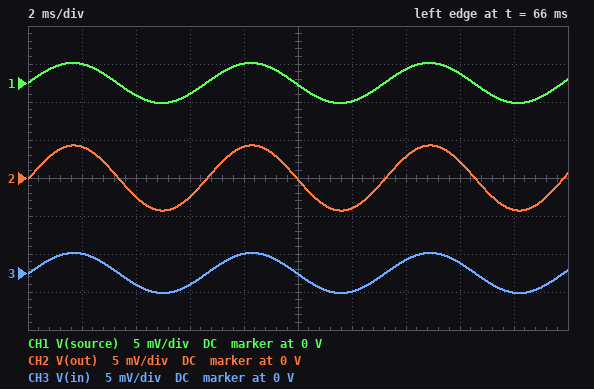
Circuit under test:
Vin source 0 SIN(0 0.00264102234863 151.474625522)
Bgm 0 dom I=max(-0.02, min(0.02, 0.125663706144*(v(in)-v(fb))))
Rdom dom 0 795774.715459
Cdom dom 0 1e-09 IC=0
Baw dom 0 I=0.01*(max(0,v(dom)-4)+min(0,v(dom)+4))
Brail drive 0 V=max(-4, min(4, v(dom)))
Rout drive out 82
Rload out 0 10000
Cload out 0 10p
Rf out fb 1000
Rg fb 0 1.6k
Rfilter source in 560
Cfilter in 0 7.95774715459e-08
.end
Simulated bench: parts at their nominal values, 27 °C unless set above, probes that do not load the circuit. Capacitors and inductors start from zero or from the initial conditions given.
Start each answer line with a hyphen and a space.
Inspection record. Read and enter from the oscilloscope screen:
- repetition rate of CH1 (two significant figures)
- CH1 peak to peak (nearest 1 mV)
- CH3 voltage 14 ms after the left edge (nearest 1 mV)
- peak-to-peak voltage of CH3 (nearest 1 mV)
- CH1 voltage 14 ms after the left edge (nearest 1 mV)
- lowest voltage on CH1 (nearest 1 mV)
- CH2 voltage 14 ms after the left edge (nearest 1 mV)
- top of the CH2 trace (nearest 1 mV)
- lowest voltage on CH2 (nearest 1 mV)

- 150 Hz
- 5 mV
- 2 mV
- 5 mV
- 2 mV
- -3 mV
- 3 mV
- 4 mV
- -4 mV
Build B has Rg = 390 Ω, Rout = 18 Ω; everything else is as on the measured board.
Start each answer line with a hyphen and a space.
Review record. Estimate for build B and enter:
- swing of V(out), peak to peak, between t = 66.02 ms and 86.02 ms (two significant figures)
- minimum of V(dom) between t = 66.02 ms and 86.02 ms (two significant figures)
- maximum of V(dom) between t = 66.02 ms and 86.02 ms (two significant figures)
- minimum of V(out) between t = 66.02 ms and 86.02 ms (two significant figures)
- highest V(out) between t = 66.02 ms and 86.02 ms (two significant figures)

- 19 mV
- -9.5 mV
- 9.5 mV
- -9.4 mV
- 9.4 mV
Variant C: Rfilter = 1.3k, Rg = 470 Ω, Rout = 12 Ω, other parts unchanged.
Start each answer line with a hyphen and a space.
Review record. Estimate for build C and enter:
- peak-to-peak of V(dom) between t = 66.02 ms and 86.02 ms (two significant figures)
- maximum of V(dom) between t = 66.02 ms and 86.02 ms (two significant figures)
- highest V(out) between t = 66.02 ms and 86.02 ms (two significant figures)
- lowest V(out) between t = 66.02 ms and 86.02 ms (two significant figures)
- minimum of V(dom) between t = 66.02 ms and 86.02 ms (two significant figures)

- 17 mV
- 8.3 mV
- 8.2 mV
- -8.2 mV
- -8.3 mV
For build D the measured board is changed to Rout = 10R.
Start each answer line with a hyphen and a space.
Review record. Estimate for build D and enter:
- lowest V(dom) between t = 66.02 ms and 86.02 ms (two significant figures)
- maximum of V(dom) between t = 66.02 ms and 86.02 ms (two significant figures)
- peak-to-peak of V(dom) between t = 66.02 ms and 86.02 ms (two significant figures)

- -4.3 mV
- 4.3 mV
- 8.6 mV
